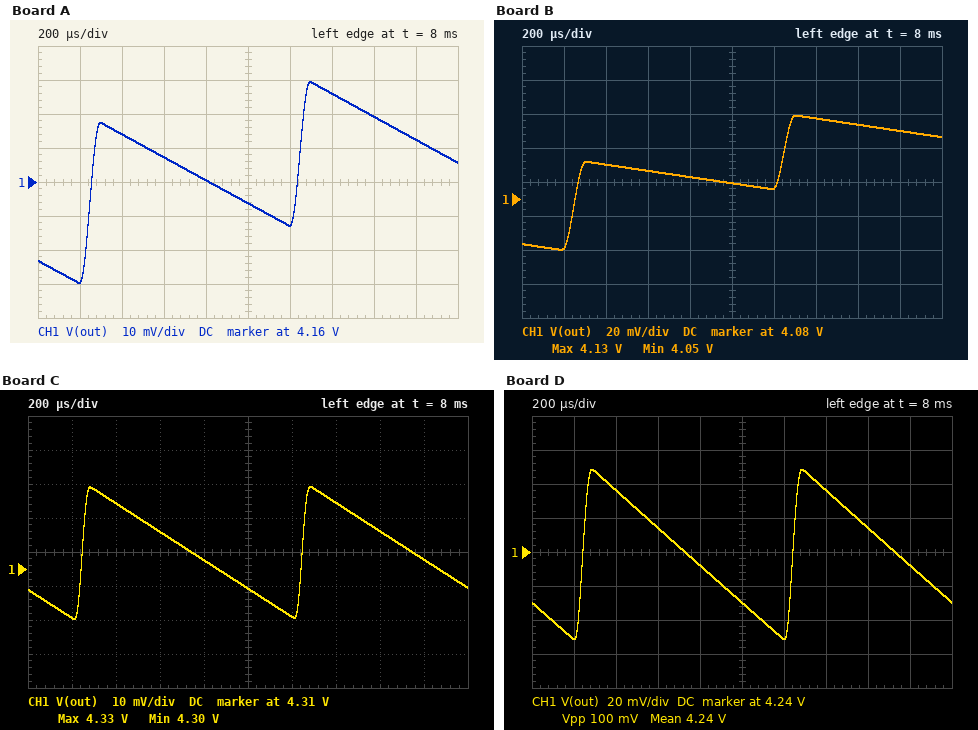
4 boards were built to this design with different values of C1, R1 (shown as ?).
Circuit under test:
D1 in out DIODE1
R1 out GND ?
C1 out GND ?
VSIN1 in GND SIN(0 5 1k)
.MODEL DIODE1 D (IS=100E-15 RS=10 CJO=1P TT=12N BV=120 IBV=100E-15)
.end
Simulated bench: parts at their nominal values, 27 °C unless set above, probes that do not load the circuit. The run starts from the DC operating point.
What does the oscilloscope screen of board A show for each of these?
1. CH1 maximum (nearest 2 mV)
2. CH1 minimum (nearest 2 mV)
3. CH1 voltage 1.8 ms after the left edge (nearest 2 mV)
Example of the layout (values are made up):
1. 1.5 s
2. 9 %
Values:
1. 4.190 V
2. 4.130 V
3. 4.172 V
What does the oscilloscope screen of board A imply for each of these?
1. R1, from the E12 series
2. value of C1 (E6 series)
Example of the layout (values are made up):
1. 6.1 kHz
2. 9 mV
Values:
1. 5.6 kΩ
2. 22 µF
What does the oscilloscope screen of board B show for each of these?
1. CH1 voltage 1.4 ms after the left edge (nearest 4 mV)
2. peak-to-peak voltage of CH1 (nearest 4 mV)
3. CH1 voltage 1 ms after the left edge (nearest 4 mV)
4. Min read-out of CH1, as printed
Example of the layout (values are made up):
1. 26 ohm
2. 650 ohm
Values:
1. 4.128 V
2. 80 mV
3. 4.088 V
4. 4.05 V
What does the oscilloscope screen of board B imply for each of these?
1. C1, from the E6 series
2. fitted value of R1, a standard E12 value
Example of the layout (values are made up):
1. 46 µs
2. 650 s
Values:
1. 33 µF
2. 6.8 kΩ
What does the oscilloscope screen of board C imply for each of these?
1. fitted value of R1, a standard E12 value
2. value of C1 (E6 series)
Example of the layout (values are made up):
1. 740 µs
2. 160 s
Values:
1. 22 kΩ
2. 4.7 µF
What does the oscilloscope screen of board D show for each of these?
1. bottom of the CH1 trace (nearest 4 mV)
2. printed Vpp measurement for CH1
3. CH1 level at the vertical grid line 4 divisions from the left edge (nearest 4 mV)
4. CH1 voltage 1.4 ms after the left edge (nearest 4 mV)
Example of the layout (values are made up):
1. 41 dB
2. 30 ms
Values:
1. 4.188 V
2. 100 mV
3. 4.232 V
4. 4.276 V
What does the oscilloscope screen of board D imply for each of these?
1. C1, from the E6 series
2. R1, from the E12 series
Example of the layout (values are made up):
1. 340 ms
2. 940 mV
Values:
1. 4.7 µF
2. 8.2 kΩ
